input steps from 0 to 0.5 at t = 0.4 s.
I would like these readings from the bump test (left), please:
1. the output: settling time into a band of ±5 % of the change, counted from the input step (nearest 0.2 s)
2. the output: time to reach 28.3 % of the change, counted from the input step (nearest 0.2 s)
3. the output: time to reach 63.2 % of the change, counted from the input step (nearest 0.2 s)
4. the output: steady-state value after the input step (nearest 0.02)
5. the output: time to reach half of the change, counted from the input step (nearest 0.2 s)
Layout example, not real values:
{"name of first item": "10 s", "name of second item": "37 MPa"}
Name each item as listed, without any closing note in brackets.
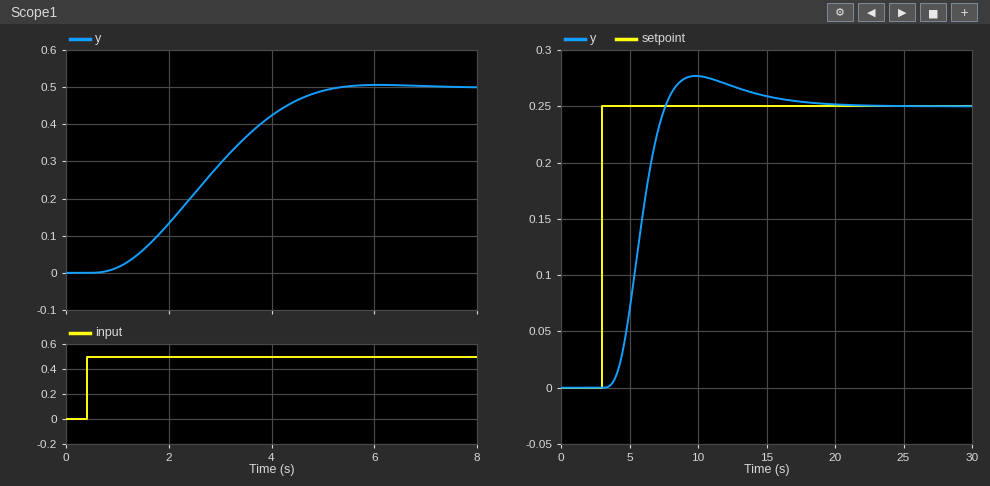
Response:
{"the output: settling time into a band of ±5 % of the change, counted from the input step": "4.2 s", "the output: time to reach 28.3 % of the change, counted from the input step": "1.6 s", "the output: time to reach 63.2 % of the change, counted from the input step": "2.8 s", "the output: steady-state value after the input step": "0.50", "the output: time to reach half of the change, counted from the input step": "2.4 s"}
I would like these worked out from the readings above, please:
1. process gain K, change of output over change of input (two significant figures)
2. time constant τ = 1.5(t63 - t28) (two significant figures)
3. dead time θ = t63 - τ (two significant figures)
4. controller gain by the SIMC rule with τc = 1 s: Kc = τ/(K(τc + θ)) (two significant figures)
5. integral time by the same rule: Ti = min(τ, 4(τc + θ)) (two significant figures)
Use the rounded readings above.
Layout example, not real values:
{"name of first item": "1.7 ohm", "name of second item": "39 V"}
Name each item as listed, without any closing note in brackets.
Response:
{"process gain K, change of output over change of input": "1.0", "time constant τ = 1.5(t63 - t28)": "1.8 s", "dead time θ = t63 - τ": "1.0 s", "controller gain by the SIMC rule with τc = 1 s: Kc = τ/(K(τc + θ))": "0.90", "integral time by the same rule: Ti = min(τ, 4(τc + θ))": "1.8 s"}
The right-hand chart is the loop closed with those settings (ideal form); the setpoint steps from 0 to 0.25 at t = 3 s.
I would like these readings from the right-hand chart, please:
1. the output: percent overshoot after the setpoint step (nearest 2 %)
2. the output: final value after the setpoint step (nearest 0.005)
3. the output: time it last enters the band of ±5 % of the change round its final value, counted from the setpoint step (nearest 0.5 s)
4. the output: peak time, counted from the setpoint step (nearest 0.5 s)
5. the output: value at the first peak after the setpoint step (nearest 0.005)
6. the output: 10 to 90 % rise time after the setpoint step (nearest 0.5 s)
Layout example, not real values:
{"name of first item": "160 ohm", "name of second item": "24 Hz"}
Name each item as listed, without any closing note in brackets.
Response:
{"the output: percent overshoot after the setpoint step": "10 %", "the output: final value after the setpoint step": "0.250", "the output: time it last enters the band of ±5 % of the change round its final value, counted from the setpoint step": "11.0 s", "the output: peak time, counted from the setpoint step": "7.0 s", "the output: value at the first peak after the setpoint step": "0.275", "the output: 10 to 90 % rise time after the setpoint step": "2.5 s"}
